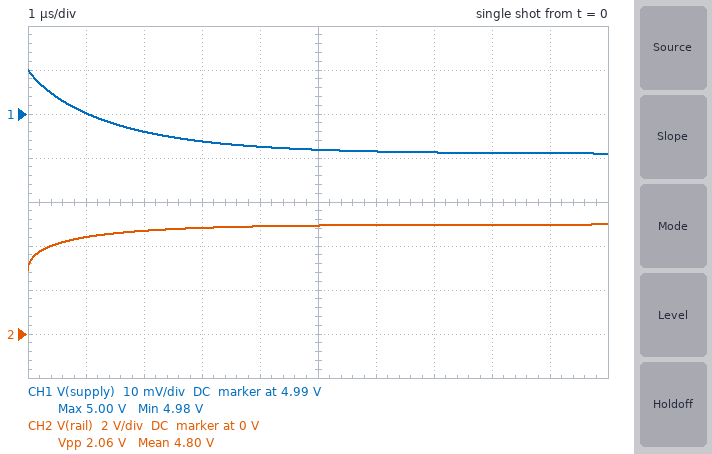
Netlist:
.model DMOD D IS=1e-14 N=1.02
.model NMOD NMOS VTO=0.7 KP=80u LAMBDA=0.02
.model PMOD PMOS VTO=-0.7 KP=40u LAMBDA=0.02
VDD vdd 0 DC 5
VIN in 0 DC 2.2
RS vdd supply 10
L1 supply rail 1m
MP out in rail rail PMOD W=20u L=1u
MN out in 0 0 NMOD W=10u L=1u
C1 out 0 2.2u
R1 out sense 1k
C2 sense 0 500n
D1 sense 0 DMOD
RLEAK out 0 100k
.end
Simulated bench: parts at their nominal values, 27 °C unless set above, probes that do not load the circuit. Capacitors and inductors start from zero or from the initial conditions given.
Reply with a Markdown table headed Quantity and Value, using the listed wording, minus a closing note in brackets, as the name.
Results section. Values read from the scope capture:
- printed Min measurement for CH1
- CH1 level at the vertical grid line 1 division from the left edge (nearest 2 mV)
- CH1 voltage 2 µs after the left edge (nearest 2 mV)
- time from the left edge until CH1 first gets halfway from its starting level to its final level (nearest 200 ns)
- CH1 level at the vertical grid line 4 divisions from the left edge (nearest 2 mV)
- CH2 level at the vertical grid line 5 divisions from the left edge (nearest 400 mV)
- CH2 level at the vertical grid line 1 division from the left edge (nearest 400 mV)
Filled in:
| Quantity | Value |
|---|---|
| printed Min measurement for CH1 | 4.98 V |
| CH1 level at the vertical grid line 1 division from the left edge | 4.990 V |
| CH1 voltage 2 µs after the left edge | 4.986 V |
| time from the left edge until CH1 first gets halfway from its starting level to its final level | 1.0 µs |
| CH1 level at the vertical grid line 4 divisions from the left edge | 4.982 V |
| CH2 level at the vertical grid line 5 divisions from the left edge | 4.8 V |
| CH2 level at the vertical grid line 1 division from the left edge | 4.4 V |
